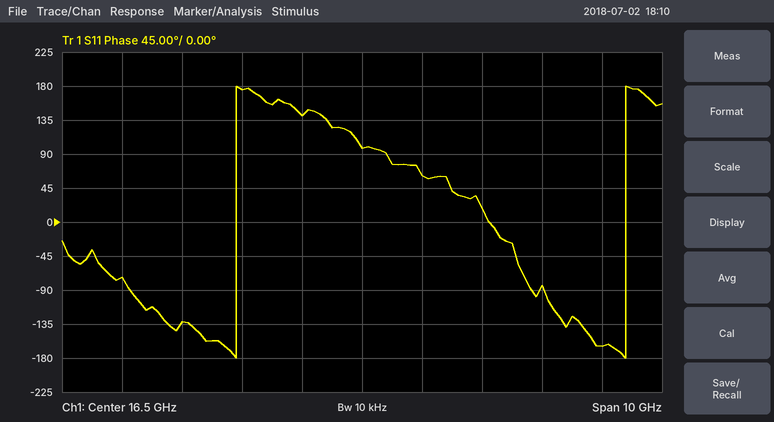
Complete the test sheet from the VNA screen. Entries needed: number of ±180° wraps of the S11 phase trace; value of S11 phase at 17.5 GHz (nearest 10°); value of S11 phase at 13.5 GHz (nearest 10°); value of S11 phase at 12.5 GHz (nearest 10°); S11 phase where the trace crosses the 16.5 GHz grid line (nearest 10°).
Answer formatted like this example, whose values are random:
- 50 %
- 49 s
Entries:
- 2
- 60°
- -130°
- -70°
- 100°
